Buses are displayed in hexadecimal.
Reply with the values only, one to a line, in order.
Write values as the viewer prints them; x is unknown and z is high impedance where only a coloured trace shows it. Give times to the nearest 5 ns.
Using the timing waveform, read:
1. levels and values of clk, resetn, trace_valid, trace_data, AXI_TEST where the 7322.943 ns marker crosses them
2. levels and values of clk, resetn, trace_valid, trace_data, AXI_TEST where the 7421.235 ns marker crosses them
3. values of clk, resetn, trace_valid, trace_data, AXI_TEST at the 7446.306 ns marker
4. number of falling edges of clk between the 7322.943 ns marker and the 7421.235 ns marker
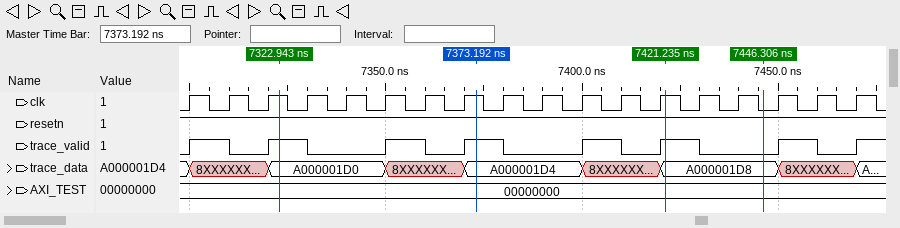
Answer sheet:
clk=1, resetn=1, trace_valid=1, trace_data=A000001D0, AXI_TEST=00000000
clk=1, resetn=1, trace_valid=1, trace_data=A000001D8, AXI_TEST=00000000
clk=0, resetn=1, trace_valid=0, trace_data=A000001D8, AXI_TEST=00000000
10
